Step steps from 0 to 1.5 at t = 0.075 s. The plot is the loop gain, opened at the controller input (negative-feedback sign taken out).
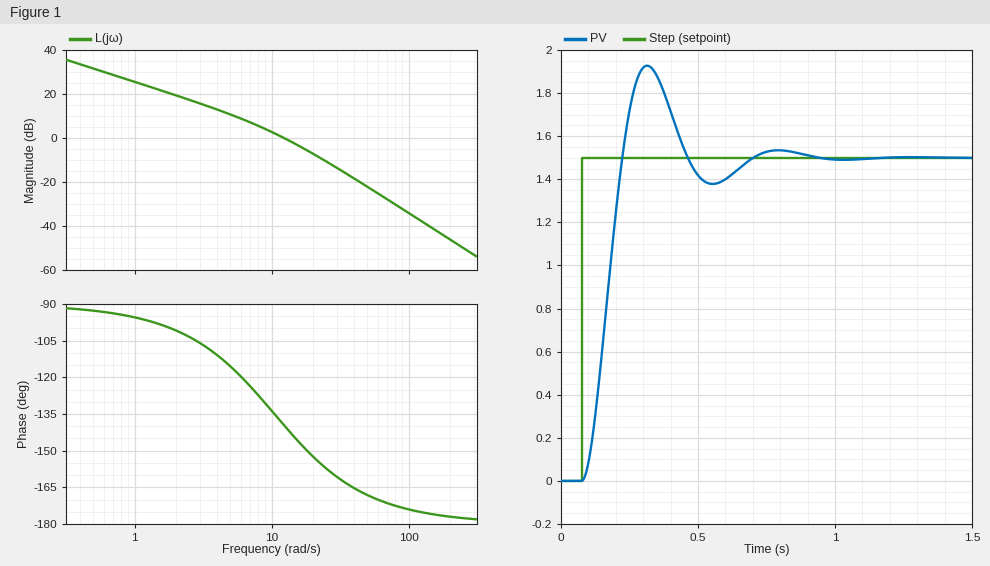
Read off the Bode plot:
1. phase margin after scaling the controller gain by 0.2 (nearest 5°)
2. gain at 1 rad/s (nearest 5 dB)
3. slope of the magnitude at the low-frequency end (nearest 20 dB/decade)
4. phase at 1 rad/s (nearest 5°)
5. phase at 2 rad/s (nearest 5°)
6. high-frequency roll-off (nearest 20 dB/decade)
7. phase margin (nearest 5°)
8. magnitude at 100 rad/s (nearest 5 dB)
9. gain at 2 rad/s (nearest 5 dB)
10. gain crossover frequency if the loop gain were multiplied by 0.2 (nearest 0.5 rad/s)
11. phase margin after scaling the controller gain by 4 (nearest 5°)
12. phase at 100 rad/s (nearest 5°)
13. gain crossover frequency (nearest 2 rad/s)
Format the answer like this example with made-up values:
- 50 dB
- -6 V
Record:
- 70°
- 25 dB
- -20 dB/decade
- -95°
- -100°
- -40 dB/decade
- 40°
- -35 dB
- 20 dB
- 3.5 rad/s
- 20°
- -175°
- 12 rad/s
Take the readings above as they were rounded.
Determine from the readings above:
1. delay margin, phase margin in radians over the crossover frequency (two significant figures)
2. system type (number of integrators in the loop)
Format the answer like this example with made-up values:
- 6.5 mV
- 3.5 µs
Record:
- 0.058 s
- 1
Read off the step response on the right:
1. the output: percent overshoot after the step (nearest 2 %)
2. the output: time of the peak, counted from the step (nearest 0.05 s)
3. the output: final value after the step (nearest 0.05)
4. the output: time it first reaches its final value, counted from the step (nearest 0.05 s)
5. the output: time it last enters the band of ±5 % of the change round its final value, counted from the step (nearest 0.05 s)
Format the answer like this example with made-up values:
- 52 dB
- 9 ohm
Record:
- 28 %
- 0.25 s
- 1.50
- 0.15 s
- 0.55 s
